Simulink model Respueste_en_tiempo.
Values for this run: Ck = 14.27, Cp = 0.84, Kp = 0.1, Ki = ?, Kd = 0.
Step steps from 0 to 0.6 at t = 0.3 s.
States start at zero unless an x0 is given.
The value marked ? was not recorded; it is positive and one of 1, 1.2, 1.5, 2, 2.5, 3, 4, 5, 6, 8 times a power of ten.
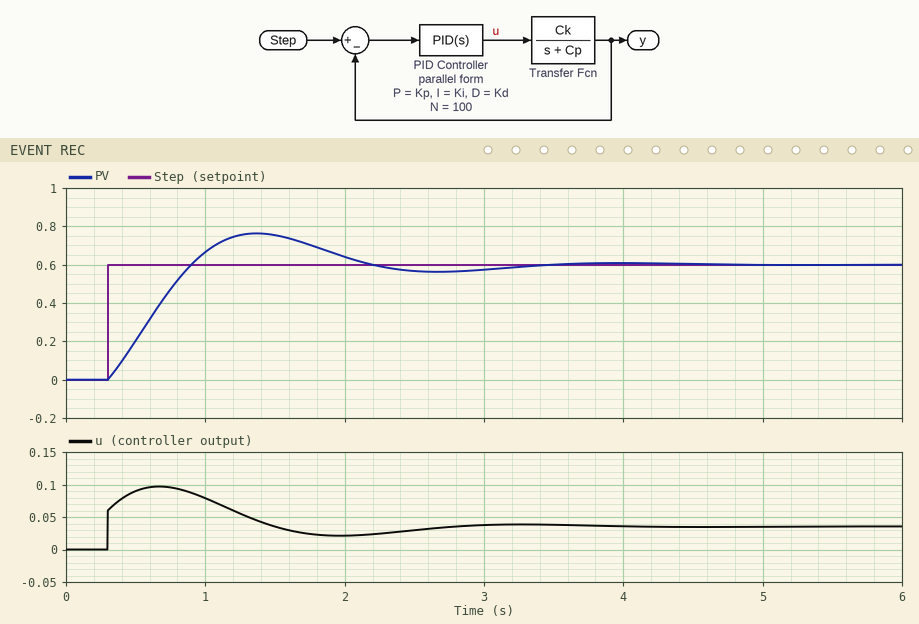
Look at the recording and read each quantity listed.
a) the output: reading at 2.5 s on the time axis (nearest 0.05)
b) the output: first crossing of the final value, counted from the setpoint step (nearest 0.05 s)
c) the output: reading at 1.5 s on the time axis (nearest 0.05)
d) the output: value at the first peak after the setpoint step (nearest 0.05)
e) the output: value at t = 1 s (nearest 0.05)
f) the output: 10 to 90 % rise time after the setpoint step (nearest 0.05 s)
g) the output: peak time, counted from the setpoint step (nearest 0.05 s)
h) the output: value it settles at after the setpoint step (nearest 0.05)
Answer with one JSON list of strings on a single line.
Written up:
["0.55", "0.60 s", "0.75", "0.75", "0.65", "0.45 s", "1.05 s", "0.60"]
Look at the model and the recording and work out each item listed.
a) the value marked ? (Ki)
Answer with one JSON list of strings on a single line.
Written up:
["0.5"]
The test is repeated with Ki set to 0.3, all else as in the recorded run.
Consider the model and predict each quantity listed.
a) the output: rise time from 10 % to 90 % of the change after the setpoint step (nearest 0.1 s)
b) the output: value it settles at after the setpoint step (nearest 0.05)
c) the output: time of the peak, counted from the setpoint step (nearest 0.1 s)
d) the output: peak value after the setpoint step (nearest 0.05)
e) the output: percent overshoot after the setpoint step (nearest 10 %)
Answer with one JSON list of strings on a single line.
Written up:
["0.6 s", "0.60", "1.4 s", "0.70", "20 %"]
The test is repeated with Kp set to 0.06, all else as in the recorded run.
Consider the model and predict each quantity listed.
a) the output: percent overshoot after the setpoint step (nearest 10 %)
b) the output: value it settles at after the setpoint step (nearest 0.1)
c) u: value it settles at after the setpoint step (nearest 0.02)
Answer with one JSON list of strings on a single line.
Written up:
["40 %", "0.6", "0.04"]
